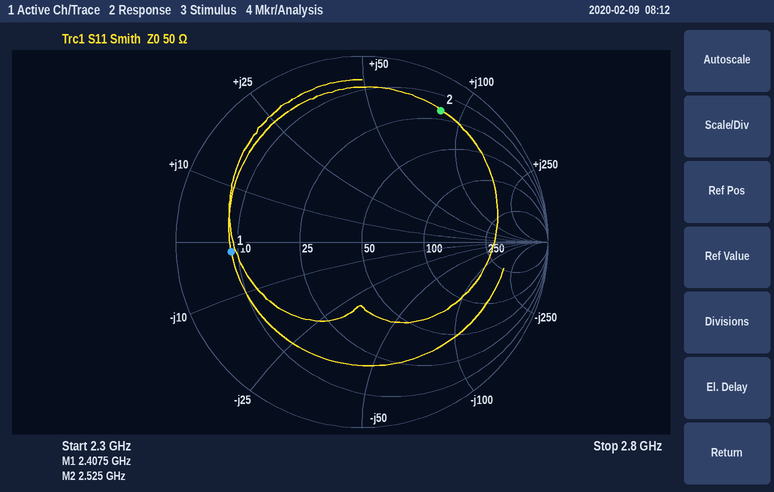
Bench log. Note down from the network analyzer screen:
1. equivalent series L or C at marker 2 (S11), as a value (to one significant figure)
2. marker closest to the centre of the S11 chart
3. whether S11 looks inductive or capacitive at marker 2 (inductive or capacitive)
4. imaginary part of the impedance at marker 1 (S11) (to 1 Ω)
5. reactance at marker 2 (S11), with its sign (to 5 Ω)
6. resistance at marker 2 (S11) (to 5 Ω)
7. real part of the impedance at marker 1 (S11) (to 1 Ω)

5 nH
marker 1
inductive
-2 Ω
+85 Ω
20 Ω
9 Ω
